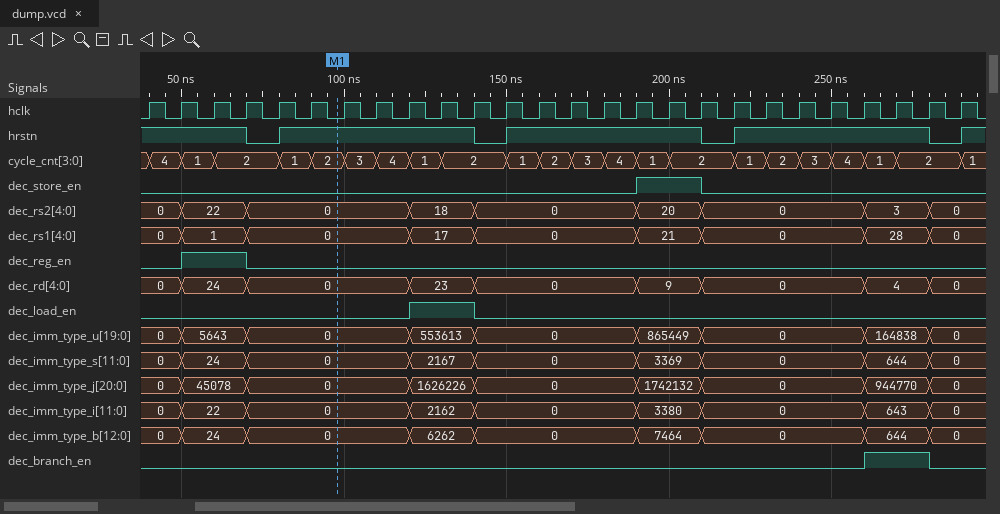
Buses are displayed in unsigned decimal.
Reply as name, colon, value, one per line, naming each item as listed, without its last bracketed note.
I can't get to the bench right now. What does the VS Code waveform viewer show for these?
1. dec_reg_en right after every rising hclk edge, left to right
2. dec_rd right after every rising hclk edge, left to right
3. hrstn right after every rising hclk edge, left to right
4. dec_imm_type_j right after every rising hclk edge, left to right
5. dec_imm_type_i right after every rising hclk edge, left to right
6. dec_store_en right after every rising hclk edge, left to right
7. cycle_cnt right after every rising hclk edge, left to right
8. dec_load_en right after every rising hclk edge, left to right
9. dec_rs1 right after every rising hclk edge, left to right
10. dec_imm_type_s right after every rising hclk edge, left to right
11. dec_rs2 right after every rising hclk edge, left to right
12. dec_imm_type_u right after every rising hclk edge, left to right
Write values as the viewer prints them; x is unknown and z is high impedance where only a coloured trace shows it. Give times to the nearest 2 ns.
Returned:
dec_reg_en right after every rising hclk edge, left to right: 0 1 1 0 0 0 0 0 0 0 0 0 0 0 0 0 0 0 0 0 0 0 0 0 0 0
dec_rd right after every rising hclk edge, left to right: 0, 24, 24, 0, 0, 0, 0, 0, 23, 23, 0, 0, 0, 0, 0, 9, 9, 0, 0, 0, 0, 0, 4, 4, 0, 0
hrstn right after every rising hclk edge, left to right: 1 1 1 0 1 1 1 1 1 1 0 1 1 1 1 1 1 0 1 1 1 1 1 1 0 1
dec_imm_type_j right after every rising hclk edge, left to right: 0, 45078, 45078, 0, 0, 0, 0, 0, 1626226, 1626226, 0, 0, 0, 0, 0, 1742132, 1742132, 0, 0, 0, 0, 0, 944770, 944770, 0, 0
dec_imm_type_i right after every rising hclk edge, left to right: 0, 22, 22, 0, 0, 0, 0, 0, 2162, 2162, 0, 0, 0, 0, 0, 3380, 3380, 0, 0, 0, 0, 0, 643, 643, 0, 0
dec_store_en right after every rising hclk edge, left to right: 0 0 0 0 0 0 0 0 0 0 0 0 0 0 0 1 1 0 0 0 0 0 0 0 0 0
cycle_cnt right after every rising hclk edge, left to right: 4, 1, 2, 2, 1, 2, 3, 4, 1, 2, 2, 1, 2, 3, 4, 1, 2, 2, 1, 2, 3, 4, 1, 2, 2, 1
dec_load_en right after every rising hclk edge, left to right: 0 0 0 0 0 0 0 0 1 1 0 0 0 0 0 0 0 0 0 0 0 0 0 0 0 0
dec_rs1 right after every rising hclk edge, left to right: 0, 1, 1, 0, 0, 0, 0, 0, 17, 17, 0, 0, 0, 0, 0, 21, 21, 0, 0, 0, 0, 0, 28, 28, 0, 0
dec_imm_type_s right after every rising hclk edge, left to right: 0, 24, 24, 0, 0, 0, 0, 0, 2167, 2167, 0, 0, 0, 0, 0, 3369, 3369, 0, 0, 0, 0, 0, 644, 644, 0, 0
dec_rs2 right after every rising hclk edge, left to right: 0, 22, 22, 0, 0, 0, 0, 0, 18, 18, 0, 0, 0, 0, 0, 20, 20, 0, 0, 0, 0, 0, 3, 3, 0, 0
dec_imm_type_u right after every rising hclk edge, left to right: 0, 5643, 5643, 0, 0, 0, 0, 0, 553613, 553613, 0, 0, 0, 0, 0, 865449, 865449, 0, 0, 0, 0, 0, 164838, 164838, 0, 0
